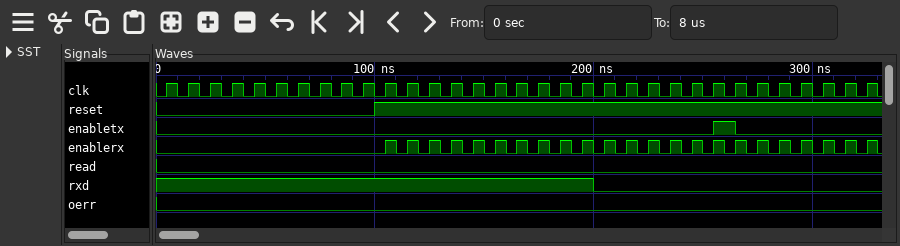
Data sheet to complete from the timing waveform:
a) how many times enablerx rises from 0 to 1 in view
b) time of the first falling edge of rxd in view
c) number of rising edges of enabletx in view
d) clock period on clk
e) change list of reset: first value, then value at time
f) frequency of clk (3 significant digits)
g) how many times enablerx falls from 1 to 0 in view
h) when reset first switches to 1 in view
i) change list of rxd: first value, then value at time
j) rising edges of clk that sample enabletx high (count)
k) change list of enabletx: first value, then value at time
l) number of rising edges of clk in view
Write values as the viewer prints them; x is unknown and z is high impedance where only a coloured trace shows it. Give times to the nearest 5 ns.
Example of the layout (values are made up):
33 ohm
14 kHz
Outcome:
23
200 ns
1
10 ns
0, 1 at 100 ns
100 MHz
23
100 ns
1, 0 at 200 ns
1
0, 1 at 255 ns, 0 at 265 ns
33
